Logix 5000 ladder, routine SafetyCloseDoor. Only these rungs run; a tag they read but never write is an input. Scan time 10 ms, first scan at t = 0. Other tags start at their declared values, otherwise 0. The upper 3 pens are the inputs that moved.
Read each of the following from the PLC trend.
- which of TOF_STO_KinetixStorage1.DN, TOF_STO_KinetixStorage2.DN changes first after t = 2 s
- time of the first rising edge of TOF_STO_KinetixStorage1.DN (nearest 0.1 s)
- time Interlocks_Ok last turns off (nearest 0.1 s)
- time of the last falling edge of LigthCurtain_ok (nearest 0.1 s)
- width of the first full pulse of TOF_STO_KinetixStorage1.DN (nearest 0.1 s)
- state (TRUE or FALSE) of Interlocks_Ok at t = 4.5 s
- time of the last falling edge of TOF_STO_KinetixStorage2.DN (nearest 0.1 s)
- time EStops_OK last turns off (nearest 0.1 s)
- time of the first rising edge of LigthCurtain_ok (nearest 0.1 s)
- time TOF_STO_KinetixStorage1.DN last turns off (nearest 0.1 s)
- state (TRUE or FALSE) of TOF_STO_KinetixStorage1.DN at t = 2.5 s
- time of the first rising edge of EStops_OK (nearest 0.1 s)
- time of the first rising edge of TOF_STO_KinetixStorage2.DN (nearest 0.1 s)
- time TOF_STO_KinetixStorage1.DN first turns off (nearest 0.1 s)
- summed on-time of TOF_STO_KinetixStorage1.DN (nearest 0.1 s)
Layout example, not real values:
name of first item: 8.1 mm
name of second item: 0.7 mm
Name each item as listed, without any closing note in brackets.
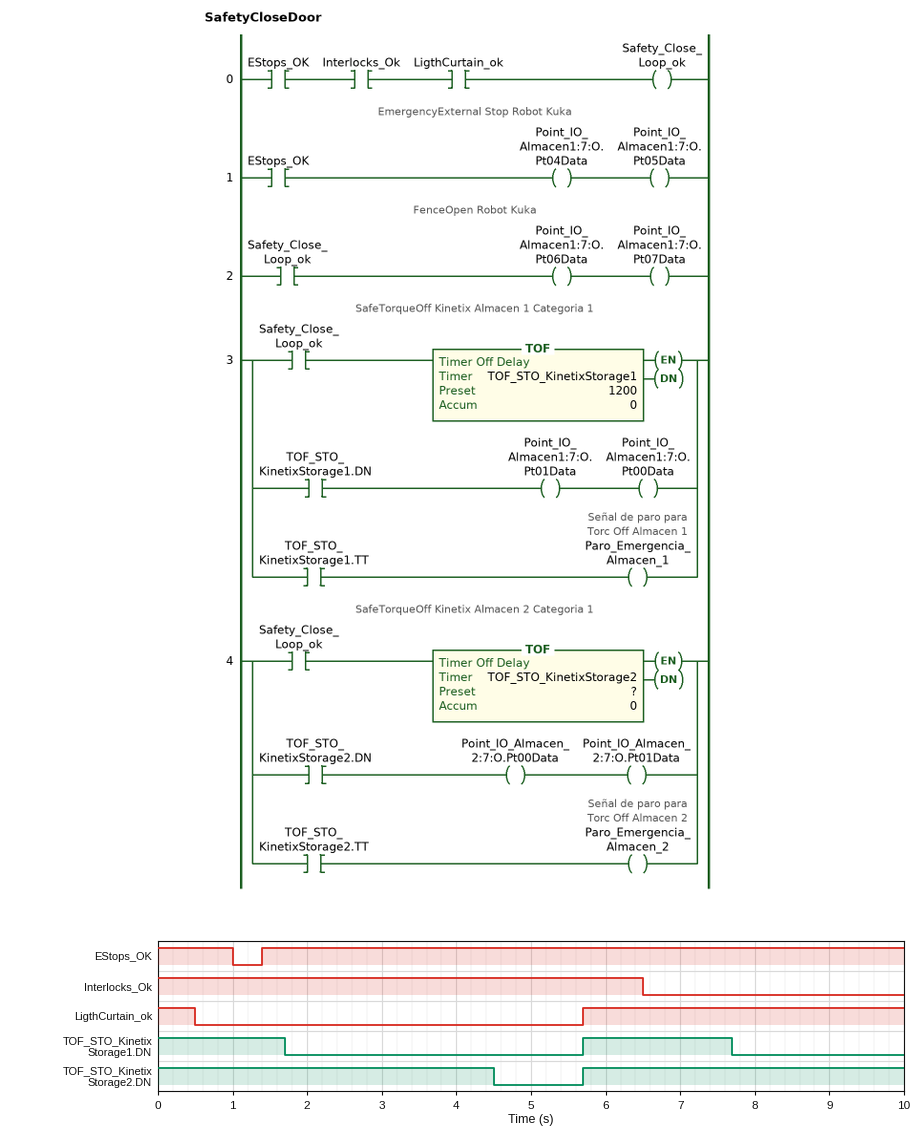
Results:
which of TOF_STO_KinetixStorage1.DN, TOF_STO_KinetixStorage2.DN changes first after t = 2 s: TOF_STO_KinetixStorage2.DN
time of the first rising edge of TOF_STO_KinetixStorage1.DN: 5.7 s
time Interlocks_Ok last turns off: 6.5 s
time of the last falling edge of LigthCurtain_ok: 0.5 s
width of the first full pulse of TOF_STO_KinetixStorage1.DN: 2.0 s
state (TRUE or FALSE) of Interlocks_Ok at t = 4.5 s: TRUE
time of the last falling edge of TOF_STO_KinetixStorage2.DN: 4.5 s
time EStops_OK last turns off: 1.0 s
time of the first rising edge of LigthCurtain_ok: 5.7 s
time TOF_STO_KinetixStorage1.DN last turns off: 7.7 s
state (TRUE or FALSE) of TOF_STO_KinetixStorage1.DN at t = 2.5 s: FALSE
time of the first rising edge of EStops_OK: 1.4 s
time of the first rising edge of TOF_STO_KinetixStorage2.DN: 5.7 s
time TOF_STO_KinetixStorage1.DN first turns off: 1.7 s
summed on-time of TOF_STO_KinetixStorage1.DN: 3.7 s
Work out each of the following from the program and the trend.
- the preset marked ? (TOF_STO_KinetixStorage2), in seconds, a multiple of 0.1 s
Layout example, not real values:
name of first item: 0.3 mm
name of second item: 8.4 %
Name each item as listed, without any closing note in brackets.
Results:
the preset marked ? (TOF_STO_KinetixStorage2), in seconds, a multiple of 0.1 s: 4.0 s
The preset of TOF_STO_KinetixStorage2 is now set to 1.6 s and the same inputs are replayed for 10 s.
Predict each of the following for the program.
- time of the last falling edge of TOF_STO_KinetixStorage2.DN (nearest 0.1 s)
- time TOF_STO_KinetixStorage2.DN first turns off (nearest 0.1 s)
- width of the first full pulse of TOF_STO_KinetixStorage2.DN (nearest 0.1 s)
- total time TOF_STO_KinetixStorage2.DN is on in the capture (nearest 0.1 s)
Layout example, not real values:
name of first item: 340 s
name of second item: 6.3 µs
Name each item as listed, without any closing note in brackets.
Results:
time of the last falling edge of TOF_STO_KinetixStorage2.DN: 8.1 s
time TOF_STO_KinetixStorage2.DN first turns off: 2.1 s
width of the first full pulse of TOF_STO_KinetixStorage2.DN: 2.4 s
total time TOF_STO_KinetixStorage2.DN is on in the capture: 4.5 s
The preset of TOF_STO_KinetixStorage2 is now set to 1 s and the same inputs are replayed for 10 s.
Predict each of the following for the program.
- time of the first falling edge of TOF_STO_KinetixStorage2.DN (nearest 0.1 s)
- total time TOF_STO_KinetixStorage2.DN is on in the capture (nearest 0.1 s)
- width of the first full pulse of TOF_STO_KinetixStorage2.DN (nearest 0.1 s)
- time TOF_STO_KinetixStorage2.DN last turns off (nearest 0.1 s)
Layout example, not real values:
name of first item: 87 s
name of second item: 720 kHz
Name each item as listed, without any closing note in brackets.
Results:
time of the first falling edge of TOF_STO_KinetixStorage2.DN: 1.5 s
total time TOF_STO_KinetixStorage2.DN is on in the capture: 3.3 s
width of the first full pulse of TOF_STO_KinetixStorage2.DN: 1.8 s
time TOF_STO_KinetixStorage2.DN last turns off: 7.5 s
